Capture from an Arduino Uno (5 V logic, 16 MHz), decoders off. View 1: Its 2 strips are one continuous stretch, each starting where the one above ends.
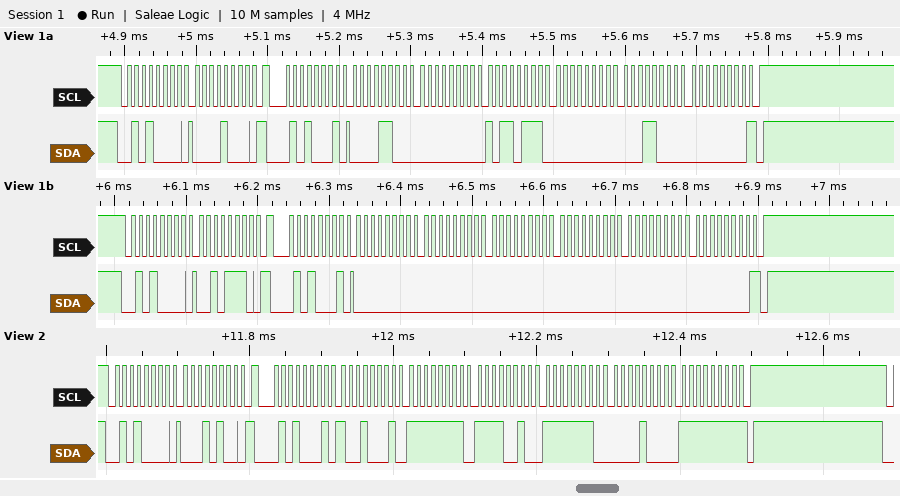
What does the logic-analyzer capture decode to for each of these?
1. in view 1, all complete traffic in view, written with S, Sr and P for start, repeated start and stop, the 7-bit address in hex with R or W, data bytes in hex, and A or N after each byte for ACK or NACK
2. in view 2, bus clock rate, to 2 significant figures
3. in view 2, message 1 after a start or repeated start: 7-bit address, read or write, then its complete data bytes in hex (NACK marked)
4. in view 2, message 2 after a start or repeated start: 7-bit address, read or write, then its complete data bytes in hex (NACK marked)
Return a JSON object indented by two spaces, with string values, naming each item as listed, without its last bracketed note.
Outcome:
{
  "in view 1, all complete traffic in view, written with S, Sr and P for start, repeated start and stop, the 7-bit address in hex with R or W, data bytes in hex, and A or N after each byte for ACK or NACK": "S 28W A 08 A Sr 28R A 0C A 00 A B7 A 00 A 18 A 00 N P S 28W A 2E A Sr 28R A 00 A 00 A 00 A 00 A 00 A 00 N P",
  "in view 2, bus clock rate, to 2 significant figures": "100 kHz",
  "in view 2, message 1 after a start or repeated start: 7-bit address, read or write, then its complete data bytes in hex": "0x28 write: 14",
  "in view 2, message 2 after a start or repeated start: 7-bit address, read or write, then its complete data bytes in hex": "0x28 read: 91 FF F2 FE 08 FF NACK"
}
